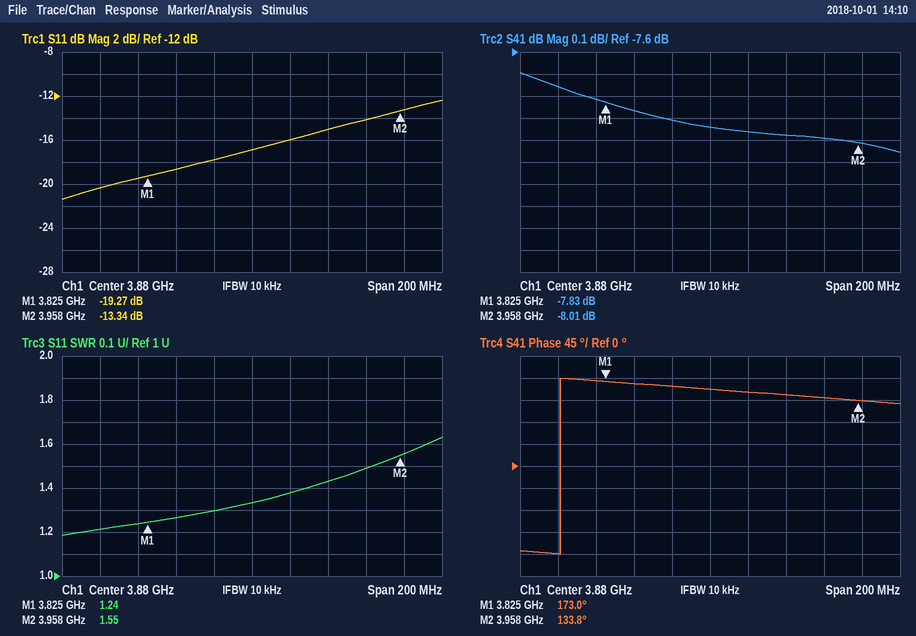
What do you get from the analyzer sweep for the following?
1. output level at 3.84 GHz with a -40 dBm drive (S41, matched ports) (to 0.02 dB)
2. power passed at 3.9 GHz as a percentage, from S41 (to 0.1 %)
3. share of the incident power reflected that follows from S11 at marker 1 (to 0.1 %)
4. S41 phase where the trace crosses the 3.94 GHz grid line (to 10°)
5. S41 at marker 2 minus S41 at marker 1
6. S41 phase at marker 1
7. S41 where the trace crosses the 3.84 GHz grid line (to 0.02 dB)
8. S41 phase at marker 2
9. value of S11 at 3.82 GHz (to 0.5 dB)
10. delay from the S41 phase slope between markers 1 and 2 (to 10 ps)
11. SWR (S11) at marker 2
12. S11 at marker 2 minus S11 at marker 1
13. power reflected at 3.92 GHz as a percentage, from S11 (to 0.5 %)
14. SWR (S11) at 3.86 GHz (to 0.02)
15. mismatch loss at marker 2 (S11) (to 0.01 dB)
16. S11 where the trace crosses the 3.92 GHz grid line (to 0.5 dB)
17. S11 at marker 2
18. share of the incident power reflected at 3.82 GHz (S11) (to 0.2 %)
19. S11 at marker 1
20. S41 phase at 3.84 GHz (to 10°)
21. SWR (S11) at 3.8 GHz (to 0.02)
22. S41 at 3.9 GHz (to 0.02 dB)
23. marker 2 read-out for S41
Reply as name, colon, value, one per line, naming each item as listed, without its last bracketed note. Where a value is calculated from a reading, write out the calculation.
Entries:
output level at 3.84 GHz with a -40 dBm drive (S41, matched ports): -40 dBm + (-7.86 dB) = -47.86 dBm
power passed at 3.9 GHz as a percentage, from S41: 10^(-7.96/10) ≈ 16.0 %
share of the incident power reflected that follows from S11 at marker 1: 10^(-19.27/10) ≈ 1.2 %
S41 phase where the trace crosses the 3.94 GHz grid line: 140°
S41 at marker 2 minus S41 at marker 1: -8.01 − (-7.83) = -0.18 dB
S41 phase at marker 1: 173.0°
S41 where the trace crosses the 3.84 GHz grid line: -7.86 dB
S41 phase at marker 2: 133.8°
value of S11 at 3.82 GHz: -19.5 dB
delay from the S41 phase slope between markers 1 and 2: −(133.8° − (173°))/(360° × 133 MHz) ≈ 819 ps, so 820 ps to the nearest 10 ps
SWR (S11) at marker 2: 1.55
S11 at marker 2 minus S11 at marker 1: -13.34 − (-19.27) = 5.93 dB
power reflected at 3.92 GHz as a percentage, from S11: 10^(-15/10) ≈ 3.16 %, so 3.0 % to the nearest 0.5 %
SWR (S11) at 3.86 GHz: 1.30
mismatch loss at marker 2 (S11): −10 log10(1 − 10^(-13.34/10)) ≈ 0.21 dB
S11 where the trace crosses the 3.92 GHz grid line: -15.0 dB
S11 at marker 2: -13.34 dB
share of the incident power reflected at 3.82 GHz (S11): 10^(-19.5/10) ≈ 1.12 %, so 1.2 % to the nearest 0.2 %
S11 at marker 1: -19.27 dB
S41 phase at 3.84 GHz: 170°
SWR (S11) at 3.8 GHz: 1.22
S41 at 3.9 GHz: -7.96 dB
marker 2 read-out for S41: -8.01 dB
